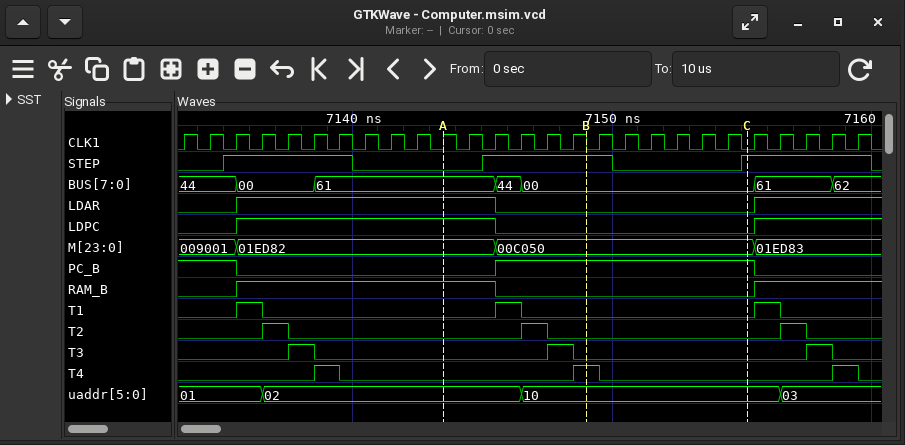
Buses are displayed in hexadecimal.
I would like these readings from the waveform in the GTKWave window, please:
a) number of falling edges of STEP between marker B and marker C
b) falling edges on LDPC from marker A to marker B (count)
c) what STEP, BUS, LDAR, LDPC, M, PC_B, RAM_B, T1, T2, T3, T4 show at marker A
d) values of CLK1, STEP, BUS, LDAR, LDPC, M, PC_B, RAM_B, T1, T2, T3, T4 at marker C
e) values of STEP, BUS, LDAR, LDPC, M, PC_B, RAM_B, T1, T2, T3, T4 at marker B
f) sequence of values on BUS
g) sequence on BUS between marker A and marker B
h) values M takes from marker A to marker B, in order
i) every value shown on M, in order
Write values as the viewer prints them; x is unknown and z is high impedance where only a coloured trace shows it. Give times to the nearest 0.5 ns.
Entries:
1
1
STEP=0, BUS=61, LDAR=1, LDPC=1, M=01ED82, PC_B=0, RAM_B=1, T1=0, T2=0, T3=0, T4=0
CLK1=0, STEP=1, BUS=00, LDAR=0, LDPC=0, M=00C050, PC_B=1, RAM_B=0, T1=0, T2=0, T3=0, T4=0
STEP=1, BUS=00, LDAR=0, LDPC=0, M=00C050, PC_B=1, RAM_B=0, T1=0, T2=0, T3=0, T4=1
44, 00, 61, 44, 00, 61, 62
61, 44, 00
01ED82, 00C050
009001, 01ED82, 00C050, 01ED83
